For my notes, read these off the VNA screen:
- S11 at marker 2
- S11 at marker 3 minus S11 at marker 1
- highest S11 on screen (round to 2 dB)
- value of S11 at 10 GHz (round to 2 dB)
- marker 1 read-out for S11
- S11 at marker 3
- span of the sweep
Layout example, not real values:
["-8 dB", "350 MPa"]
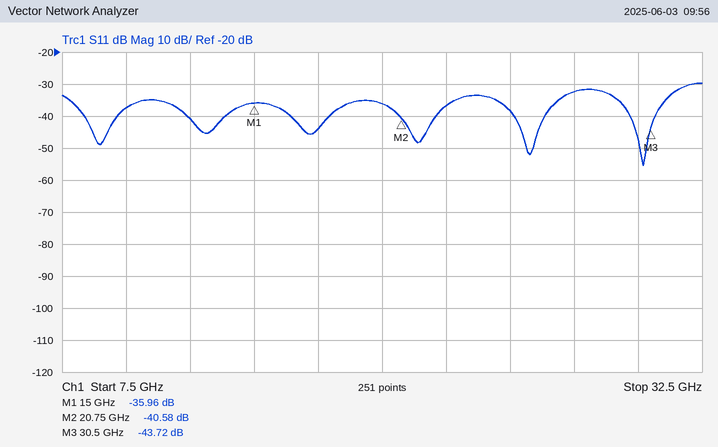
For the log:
["-40.58 dB", "-7.76 dB", "-30 dB", "-38 dB", "-35.96 dB", "-43.72 dB", "25 GHz"]
